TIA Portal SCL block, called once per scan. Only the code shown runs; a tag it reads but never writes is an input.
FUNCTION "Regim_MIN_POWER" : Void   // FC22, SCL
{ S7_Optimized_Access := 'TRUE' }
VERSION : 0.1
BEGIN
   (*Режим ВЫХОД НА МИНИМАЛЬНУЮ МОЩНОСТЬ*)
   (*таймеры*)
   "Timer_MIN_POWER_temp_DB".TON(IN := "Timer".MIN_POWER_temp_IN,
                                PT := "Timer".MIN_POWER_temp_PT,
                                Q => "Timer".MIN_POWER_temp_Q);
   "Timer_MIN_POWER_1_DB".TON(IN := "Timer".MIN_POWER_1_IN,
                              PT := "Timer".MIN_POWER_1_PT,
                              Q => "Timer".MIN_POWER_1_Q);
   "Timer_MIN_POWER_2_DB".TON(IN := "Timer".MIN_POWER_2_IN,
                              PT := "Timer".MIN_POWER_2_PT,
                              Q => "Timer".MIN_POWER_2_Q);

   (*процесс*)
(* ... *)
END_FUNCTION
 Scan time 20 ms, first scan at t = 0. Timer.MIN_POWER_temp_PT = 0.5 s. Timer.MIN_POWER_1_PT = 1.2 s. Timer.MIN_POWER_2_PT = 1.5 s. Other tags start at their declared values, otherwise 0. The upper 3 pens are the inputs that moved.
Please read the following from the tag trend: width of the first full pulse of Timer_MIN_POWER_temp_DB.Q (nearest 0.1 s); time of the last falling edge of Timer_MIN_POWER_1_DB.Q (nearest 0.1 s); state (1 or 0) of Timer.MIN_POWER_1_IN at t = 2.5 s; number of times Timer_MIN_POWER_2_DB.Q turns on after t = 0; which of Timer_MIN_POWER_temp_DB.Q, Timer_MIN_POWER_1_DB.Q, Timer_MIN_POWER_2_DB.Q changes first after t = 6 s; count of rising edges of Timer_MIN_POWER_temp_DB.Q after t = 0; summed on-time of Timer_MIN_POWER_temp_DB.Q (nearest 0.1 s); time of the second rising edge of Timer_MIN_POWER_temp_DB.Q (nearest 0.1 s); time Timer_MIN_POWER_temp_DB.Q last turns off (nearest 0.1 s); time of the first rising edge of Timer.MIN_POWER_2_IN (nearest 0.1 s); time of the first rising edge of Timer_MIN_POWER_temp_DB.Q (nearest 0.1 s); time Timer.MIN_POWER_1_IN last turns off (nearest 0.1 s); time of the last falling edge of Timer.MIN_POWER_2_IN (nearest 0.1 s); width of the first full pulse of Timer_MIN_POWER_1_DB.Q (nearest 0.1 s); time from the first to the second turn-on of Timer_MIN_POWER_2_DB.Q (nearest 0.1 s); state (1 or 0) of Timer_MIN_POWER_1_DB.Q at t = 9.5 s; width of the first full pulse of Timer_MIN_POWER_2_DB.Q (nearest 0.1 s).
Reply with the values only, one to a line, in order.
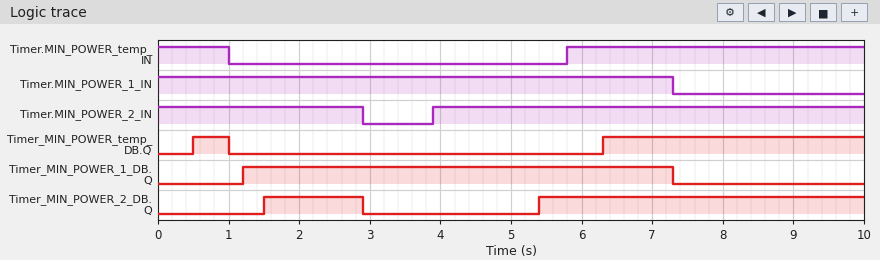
0.5 s
7.3 s
1
2
Timer_MIN_POWER_temp_DB.Q
2
4.2 s
6.3 s
1.0 s
3.9 s
0.5 s
7.3 s
2.9 s
6.1 s
3.9 s
0
1.4 s
